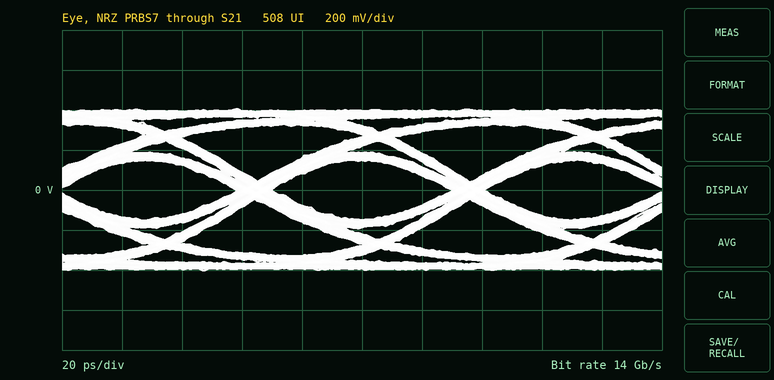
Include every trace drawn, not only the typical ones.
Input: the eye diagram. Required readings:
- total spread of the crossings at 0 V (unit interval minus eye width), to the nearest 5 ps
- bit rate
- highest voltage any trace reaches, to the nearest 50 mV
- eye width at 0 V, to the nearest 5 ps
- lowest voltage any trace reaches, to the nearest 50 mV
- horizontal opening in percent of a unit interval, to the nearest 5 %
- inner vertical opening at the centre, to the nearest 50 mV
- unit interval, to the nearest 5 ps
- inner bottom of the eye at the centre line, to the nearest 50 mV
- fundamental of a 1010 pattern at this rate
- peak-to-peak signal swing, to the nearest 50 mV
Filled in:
10 ps
14 Gb/s
400 mV
60 ps
-400 mV
85 %
300 mV
70 ps
-150 mV
7 GHz
800 mV
